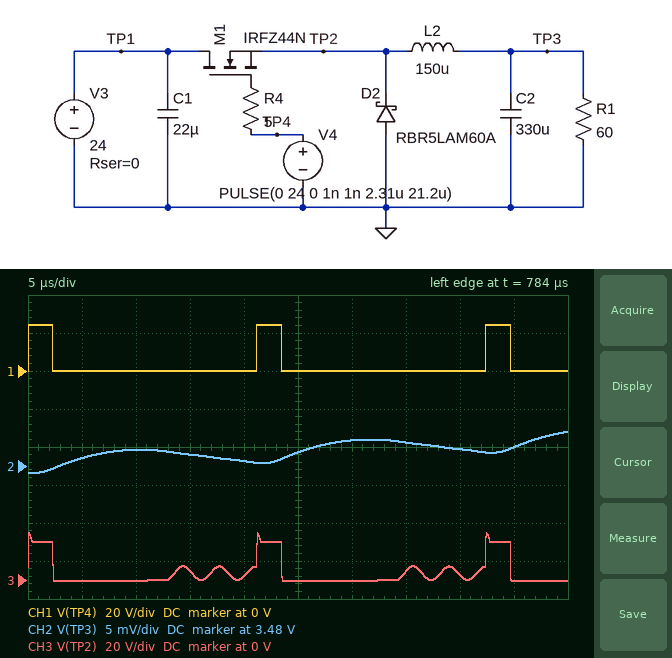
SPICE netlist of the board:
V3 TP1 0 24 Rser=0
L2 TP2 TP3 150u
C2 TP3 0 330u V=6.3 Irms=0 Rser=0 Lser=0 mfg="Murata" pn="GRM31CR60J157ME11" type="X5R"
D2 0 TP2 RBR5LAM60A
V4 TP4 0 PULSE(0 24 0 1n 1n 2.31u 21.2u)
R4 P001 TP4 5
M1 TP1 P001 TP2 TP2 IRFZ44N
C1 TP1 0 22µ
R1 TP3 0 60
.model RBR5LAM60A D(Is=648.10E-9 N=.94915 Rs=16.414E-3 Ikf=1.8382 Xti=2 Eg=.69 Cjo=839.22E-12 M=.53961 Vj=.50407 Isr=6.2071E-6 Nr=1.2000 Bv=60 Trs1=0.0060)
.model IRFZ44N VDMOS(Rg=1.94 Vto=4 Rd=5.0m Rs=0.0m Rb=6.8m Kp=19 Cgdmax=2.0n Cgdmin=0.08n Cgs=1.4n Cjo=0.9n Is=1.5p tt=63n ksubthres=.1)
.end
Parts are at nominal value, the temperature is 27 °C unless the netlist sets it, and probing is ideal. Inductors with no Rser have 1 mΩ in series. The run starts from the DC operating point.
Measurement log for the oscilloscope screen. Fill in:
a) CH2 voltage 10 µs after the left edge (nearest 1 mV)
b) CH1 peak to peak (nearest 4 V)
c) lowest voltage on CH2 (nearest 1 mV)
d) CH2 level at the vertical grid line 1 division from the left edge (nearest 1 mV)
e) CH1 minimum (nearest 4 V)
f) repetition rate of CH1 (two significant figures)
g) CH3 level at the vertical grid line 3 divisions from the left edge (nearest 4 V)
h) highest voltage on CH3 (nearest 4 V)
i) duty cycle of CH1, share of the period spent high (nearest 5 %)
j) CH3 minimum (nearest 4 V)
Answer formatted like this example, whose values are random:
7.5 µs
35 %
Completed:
3.482 V
24 V
3.479 V
3.481 V
0 V
47 kHz
4 V
24 V
10 %
0 V
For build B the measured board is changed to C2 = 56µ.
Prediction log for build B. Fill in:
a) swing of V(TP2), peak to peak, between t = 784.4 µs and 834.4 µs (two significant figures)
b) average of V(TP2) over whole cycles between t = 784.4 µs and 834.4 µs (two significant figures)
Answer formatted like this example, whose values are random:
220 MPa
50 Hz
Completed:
23 V
3.7 V
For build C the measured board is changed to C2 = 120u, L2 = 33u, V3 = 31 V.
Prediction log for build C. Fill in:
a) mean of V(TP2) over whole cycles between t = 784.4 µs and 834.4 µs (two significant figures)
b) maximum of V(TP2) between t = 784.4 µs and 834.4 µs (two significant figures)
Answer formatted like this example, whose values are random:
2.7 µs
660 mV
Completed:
4.6 V
26 V
